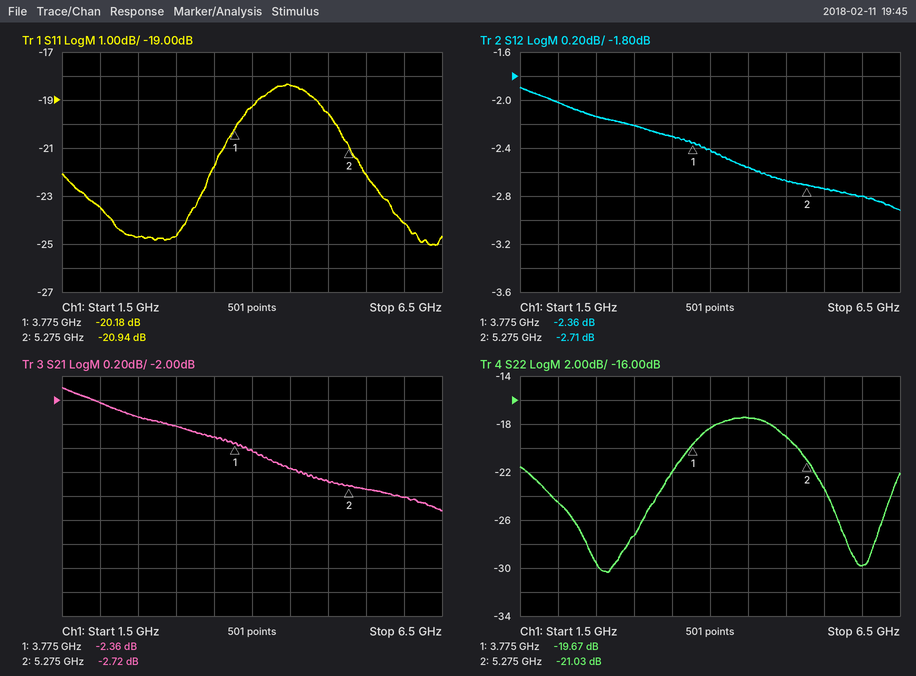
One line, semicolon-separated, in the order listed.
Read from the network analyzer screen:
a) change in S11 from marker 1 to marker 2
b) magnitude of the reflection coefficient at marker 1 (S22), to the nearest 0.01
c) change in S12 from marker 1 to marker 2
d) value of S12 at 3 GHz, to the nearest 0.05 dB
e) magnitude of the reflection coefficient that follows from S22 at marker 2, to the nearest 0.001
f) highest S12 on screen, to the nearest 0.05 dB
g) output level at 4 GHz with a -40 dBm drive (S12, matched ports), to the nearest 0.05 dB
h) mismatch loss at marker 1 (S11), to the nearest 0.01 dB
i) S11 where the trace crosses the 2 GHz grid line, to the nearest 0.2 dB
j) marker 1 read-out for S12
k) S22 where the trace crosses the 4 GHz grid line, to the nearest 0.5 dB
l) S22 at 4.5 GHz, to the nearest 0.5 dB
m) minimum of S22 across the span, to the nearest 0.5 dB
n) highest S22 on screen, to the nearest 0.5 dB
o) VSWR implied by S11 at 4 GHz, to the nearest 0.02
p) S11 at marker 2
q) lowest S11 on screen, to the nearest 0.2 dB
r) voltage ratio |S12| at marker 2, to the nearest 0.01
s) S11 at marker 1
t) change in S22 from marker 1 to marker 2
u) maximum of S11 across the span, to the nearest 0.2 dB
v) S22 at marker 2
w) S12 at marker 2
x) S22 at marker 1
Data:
-0.76 dB; 0.10; -0.35 dB; -2.20 dB; 0.089; -1.90 dB; -42.40 dBm; 0.04 dB; -23.4 dB; -2.36 dB; -18.5 dB; -17.5 dB; -30.5 dB; -17.5 dB; 1.24; -20.94 dB; -25.0 dB; 0.73; -20.18 dB; -1.36 dB; -18.4 dB; -21.03 dB; -2.71 dB; -19.67 dB
